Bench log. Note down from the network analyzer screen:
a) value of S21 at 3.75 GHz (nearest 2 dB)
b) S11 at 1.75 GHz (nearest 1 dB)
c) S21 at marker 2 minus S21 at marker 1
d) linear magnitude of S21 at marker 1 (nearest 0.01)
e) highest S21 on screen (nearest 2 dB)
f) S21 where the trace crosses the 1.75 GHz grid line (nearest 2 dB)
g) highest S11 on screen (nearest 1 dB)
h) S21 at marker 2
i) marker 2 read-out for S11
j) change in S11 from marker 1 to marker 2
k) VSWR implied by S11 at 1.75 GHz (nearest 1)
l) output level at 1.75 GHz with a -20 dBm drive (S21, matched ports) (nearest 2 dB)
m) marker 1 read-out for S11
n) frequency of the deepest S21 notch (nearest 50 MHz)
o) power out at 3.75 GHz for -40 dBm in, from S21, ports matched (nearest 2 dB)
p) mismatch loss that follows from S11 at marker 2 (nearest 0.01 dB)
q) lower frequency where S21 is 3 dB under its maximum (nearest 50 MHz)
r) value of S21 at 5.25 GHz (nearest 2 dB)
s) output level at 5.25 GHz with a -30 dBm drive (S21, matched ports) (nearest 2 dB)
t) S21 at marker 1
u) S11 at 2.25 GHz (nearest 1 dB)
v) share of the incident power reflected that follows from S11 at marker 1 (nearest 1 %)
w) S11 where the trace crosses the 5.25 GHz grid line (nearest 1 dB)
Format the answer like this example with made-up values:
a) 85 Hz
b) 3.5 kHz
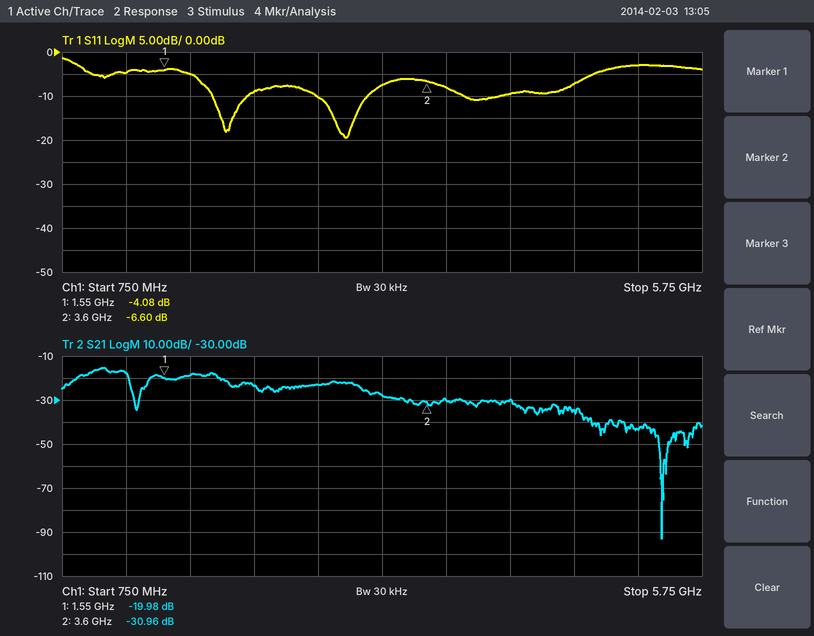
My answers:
a) -30 dB
b) -5 dB
c) -10.98 dB
d) 0.10
e) -16 dB
f) -18 dB
g) -1 dB
h) -30.96 dB
i) -6.60 dB
j) -2.52 dB
k) 4
l) -38 dBm
m) -4.08 dB
n) 5.45 GHz
o) -70 dBm
p) 1.07 dB
q) 950 MHz
r) -44 dB
s) -74 dBm
t) -19.98 dB
u) -9 dB
v) 39 %
w) -3 dB
